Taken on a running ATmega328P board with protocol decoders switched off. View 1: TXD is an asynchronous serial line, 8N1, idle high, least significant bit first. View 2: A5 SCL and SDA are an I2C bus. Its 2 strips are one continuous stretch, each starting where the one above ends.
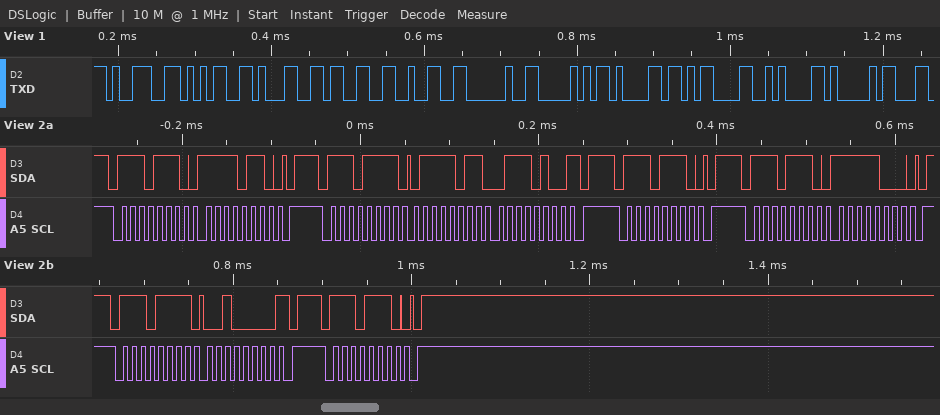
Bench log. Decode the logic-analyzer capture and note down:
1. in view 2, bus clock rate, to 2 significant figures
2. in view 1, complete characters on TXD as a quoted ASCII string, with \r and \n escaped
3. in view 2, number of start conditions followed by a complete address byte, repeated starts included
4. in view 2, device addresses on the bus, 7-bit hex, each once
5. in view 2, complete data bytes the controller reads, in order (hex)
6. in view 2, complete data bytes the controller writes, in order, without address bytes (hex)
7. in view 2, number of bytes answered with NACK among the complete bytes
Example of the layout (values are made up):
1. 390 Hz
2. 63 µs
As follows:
1. 100 kHz
2. "95132 Pa\r\nA"
3. 6
4. 0x77
5. 7B 74 20
6. F6 F8
7. 2
